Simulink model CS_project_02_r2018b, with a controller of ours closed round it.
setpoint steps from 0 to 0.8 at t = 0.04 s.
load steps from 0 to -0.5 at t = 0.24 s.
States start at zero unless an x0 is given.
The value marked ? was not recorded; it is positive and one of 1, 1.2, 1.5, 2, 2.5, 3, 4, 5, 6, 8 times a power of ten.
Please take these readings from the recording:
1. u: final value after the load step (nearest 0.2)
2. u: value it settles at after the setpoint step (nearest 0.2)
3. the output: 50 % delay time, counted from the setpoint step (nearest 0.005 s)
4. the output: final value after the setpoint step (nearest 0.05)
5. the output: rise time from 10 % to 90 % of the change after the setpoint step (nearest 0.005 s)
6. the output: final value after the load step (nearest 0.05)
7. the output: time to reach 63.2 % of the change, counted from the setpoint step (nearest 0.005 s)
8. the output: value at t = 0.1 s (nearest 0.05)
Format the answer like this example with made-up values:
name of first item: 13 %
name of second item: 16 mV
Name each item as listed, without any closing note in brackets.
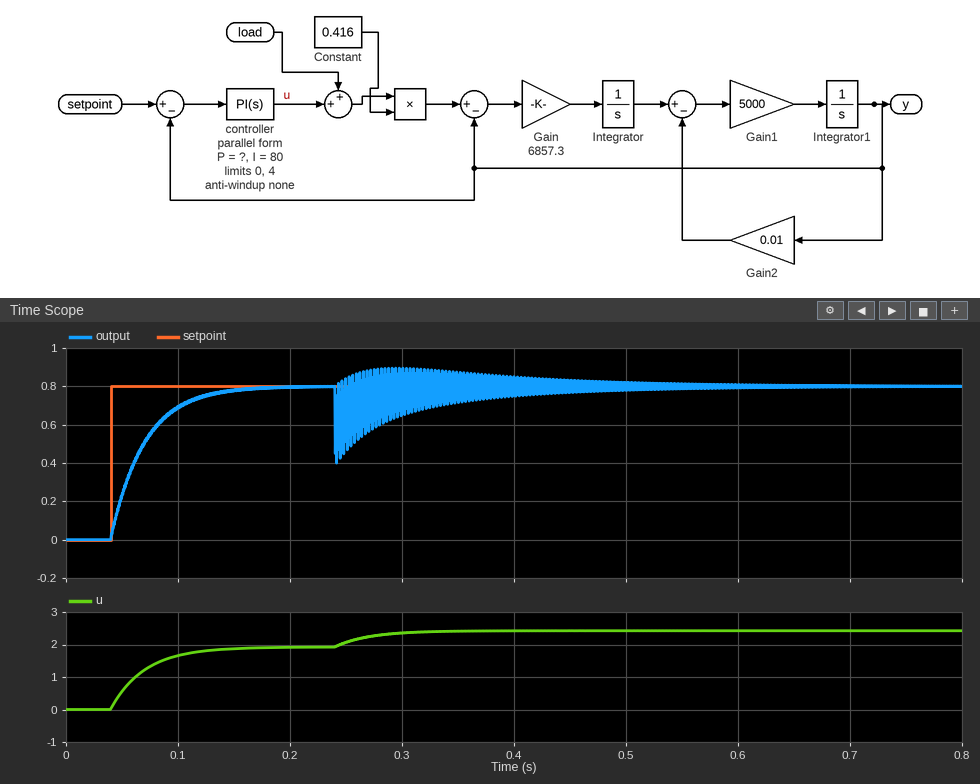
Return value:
u: final value after the load step: 2.4
u: value it settles at after the setpoint step: 2.0
the output: 50 % delay time, counted from the setpoint step: 0.020 s
the output: final value after the setpoint step: 0.80
the output: rise time from 10 % to 90 % of the change after the setpoint step: 0.065 s
the output: final value after the load step: 0.80
the output: time to reach 63.2 % of the change, counted from the setpoint step: 0.030 s
the output: value at t = 0.1 s: 0.70
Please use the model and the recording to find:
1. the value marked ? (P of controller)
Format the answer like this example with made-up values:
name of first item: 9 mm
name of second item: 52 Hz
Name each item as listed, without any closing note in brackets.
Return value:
the value marked ?: 0.03
